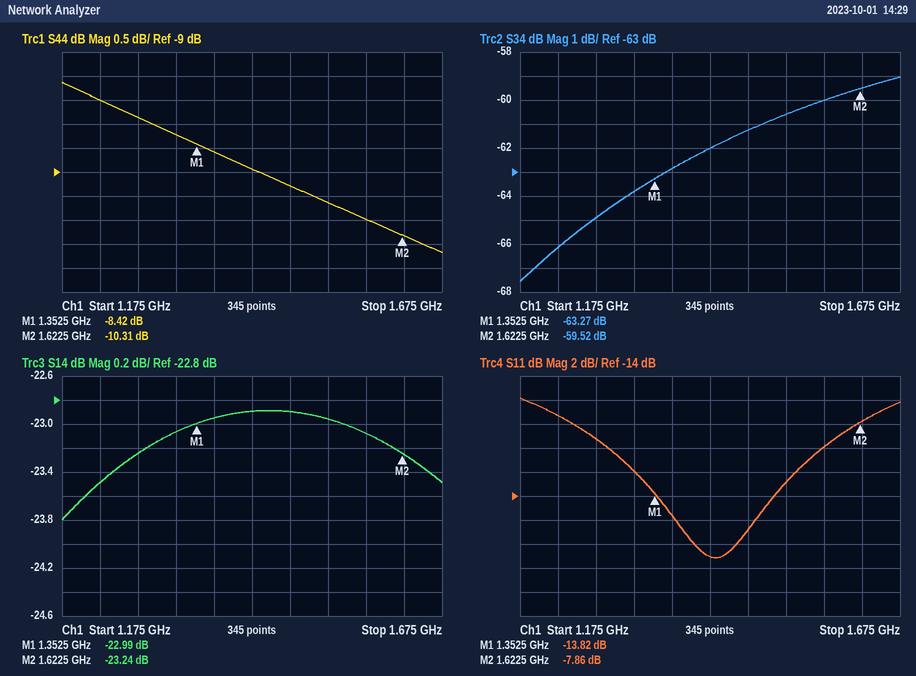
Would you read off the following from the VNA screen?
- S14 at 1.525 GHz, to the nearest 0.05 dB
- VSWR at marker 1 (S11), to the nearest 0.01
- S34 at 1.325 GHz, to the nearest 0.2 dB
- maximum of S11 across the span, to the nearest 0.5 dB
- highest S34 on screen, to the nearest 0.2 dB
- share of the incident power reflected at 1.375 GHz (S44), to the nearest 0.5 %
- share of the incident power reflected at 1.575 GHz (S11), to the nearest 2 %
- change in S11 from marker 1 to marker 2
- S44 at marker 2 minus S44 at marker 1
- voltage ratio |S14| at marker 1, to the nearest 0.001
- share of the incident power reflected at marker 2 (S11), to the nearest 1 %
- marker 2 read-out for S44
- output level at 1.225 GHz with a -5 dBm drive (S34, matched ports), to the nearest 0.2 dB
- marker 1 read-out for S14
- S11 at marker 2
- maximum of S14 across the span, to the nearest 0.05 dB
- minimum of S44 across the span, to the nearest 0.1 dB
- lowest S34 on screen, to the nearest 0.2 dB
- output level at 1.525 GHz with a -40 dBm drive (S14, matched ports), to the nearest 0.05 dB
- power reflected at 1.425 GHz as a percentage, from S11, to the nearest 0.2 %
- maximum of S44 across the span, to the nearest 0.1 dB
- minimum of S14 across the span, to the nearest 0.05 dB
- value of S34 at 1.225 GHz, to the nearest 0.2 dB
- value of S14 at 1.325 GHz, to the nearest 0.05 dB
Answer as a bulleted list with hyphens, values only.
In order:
- -22.95 dB
- 1.51
- -63.8 dB
- -6.0 dB
- -59.0 dB
- 14.0 %
- 10 %
- 5.96 dB
- -1.89 dB
- 0.071
- 16 %
- -10.31 dB
- -71.2 dBm
- -22.99 dB
- -7.86 dB
- -22.90 dB
- -10.7 dB
- -67.6 dB
- -62.95 dBm
- 1.2 %
- -7.1 dB
- -23.80 dB
- -66.2 dB
- -23.05 dB
